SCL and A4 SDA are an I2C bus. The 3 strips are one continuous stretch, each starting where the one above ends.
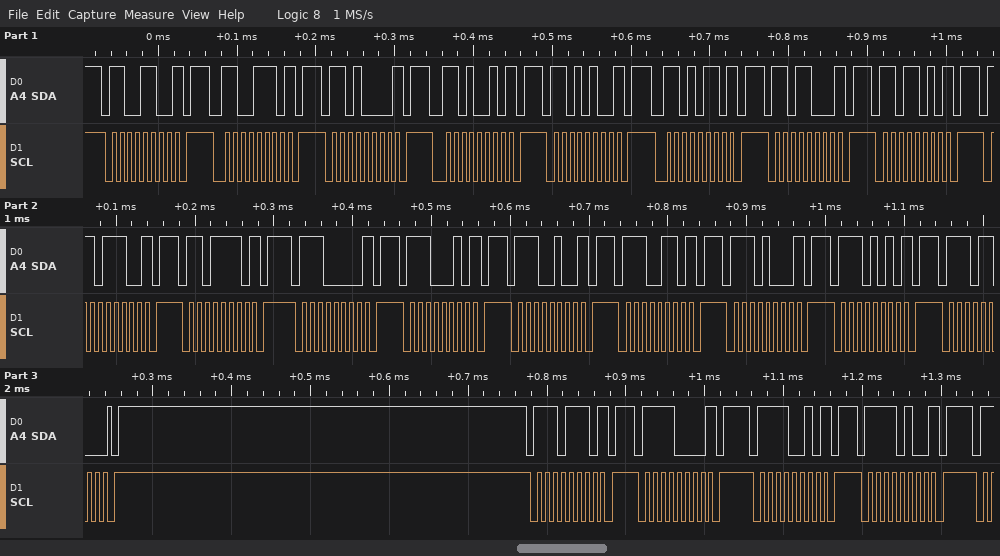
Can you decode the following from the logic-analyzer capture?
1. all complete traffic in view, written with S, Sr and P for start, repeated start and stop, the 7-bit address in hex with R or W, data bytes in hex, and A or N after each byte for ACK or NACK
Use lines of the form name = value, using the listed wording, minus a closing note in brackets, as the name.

all complete traffic in view, written with S, Sr and P for start, repeated start and stop, the 7-bit address in hex with R or W, data bytes in hex, and A or N after each byte for ACK or NACK = S 66W N P S 67W N P S 68W N P S 69W N P S 6AW N P S 6BW N P S 6CW N P S 6DW N P S 6EW N P S 6FW N P S 70W N P S 71W N P S 72W N P S 73W N P S 74W N P S 75W N P S 76W A P S 77W N P S 78W N P S 79W N P S 7AW N P
